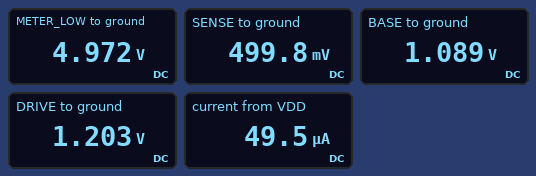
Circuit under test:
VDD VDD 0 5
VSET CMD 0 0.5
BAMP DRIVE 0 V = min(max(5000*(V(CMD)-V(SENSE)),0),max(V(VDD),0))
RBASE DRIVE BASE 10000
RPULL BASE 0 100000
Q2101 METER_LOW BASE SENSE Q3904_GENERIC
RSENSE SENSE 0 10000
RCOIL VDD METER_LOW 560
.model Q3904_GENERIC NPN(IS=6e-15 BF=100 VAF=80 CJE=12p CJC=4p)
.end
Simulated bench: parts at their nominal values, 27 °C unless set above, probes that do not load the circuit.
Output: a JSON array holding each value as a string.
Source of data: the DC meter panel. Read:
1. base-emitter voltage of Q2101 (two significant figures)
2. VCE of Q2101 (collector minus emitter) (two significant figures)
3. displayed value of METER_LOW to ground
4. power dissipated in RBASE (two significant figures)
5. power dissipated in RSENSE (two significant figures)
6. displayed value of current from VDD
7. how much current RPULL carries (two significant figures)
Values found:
["590 mV", "4.5 V", "4.972 V", "1.3 µW", "25 µW", "49.5 µA", "11 µA"]
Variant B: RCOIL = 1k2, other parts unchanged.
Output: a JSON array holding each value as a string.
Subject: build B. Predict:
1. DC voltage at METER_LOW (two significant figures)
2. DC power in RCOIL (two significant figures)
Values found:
["4.9 V", "2.9 µW"]
